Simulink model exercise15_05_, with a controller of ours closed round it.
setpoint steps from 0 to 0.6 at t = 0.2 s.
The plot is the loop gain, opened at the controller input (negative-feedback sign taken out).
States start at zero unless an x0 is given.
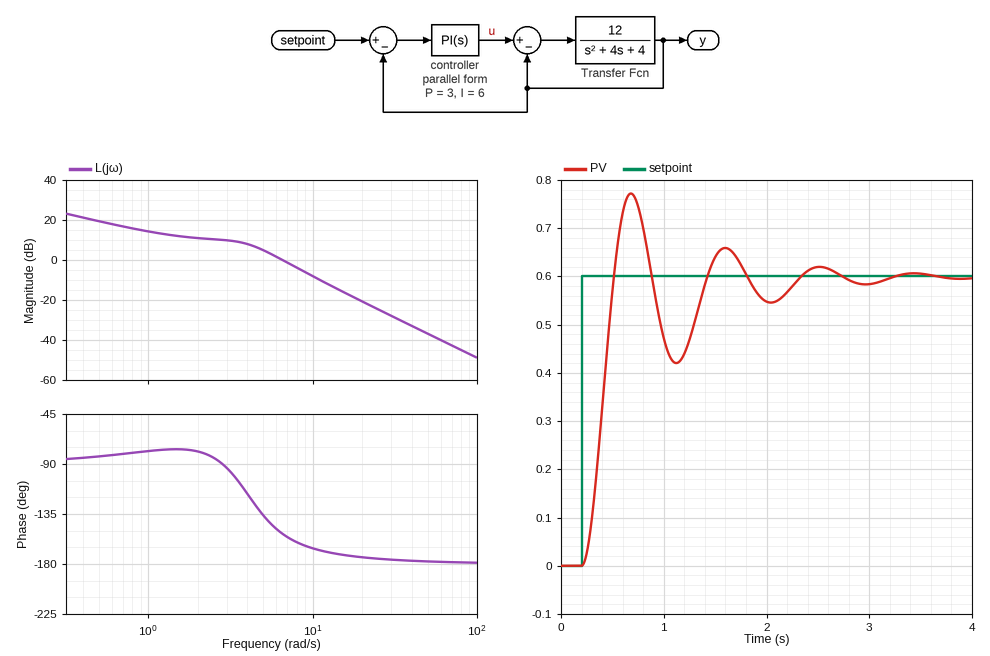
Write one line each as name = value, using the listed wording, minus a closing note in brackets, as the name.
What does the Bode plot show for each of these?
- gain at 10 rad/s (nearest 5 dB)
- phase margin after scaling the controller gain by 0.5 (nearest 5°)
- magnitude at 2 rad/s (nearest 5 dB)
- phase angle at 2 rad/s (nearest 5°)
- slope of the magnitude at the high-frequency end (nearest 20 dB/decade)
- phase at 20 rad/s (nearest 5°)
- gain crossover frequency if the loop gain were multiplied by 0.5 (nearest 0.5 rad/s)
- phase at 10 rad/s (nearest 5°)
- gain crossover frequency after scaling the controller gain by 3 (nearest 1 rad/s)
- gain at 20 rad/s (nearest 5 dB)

gain at 10 rad/s = -10 dB
phase margin after scaling the controller gain by 0.5 = 50°
magnitude at 2 rad/s = 10 dB
phase angle at 2 rad/s = -80°
slope of the magnitude at the high-frequency end = -40 dB/decade
phase at 20 rad/s = -175°
gain crossover frequency if the loop gain were multiplied by 0.5 = 4.5 rad/s
phase at 10 rad/s = -165°
gain crossover frequency after scaling the controller gain by 3 = 11 rad/s
gain at 20 rad/s = -20 dB
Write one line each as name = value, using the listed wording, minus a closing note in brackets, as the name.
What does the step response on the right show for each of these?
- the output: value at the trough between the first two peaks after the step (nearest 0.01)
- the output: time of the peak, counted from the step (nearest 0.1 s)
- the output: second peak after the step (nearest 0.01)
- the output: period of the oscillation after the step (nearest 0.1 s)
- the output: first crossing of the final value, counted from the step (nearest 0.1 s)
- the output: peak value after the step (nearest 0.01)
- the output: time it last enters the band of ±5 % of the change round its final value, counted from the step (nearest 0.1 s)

the output: value at the trough between the first two peaks after the step = 0.42
the output: time of the peak, counted from the step = 0.5 s
the output: second peak after the step = 0.66
the output: period of the oscillation after the step = 0.9 s
the output: first crossing of the final value, counted from the step = 0.3 s
the output: peak value after the step = 0.77
the output: time it last enters the band of ±5 % of the change round its final value, counted from the step = 2.0 s
